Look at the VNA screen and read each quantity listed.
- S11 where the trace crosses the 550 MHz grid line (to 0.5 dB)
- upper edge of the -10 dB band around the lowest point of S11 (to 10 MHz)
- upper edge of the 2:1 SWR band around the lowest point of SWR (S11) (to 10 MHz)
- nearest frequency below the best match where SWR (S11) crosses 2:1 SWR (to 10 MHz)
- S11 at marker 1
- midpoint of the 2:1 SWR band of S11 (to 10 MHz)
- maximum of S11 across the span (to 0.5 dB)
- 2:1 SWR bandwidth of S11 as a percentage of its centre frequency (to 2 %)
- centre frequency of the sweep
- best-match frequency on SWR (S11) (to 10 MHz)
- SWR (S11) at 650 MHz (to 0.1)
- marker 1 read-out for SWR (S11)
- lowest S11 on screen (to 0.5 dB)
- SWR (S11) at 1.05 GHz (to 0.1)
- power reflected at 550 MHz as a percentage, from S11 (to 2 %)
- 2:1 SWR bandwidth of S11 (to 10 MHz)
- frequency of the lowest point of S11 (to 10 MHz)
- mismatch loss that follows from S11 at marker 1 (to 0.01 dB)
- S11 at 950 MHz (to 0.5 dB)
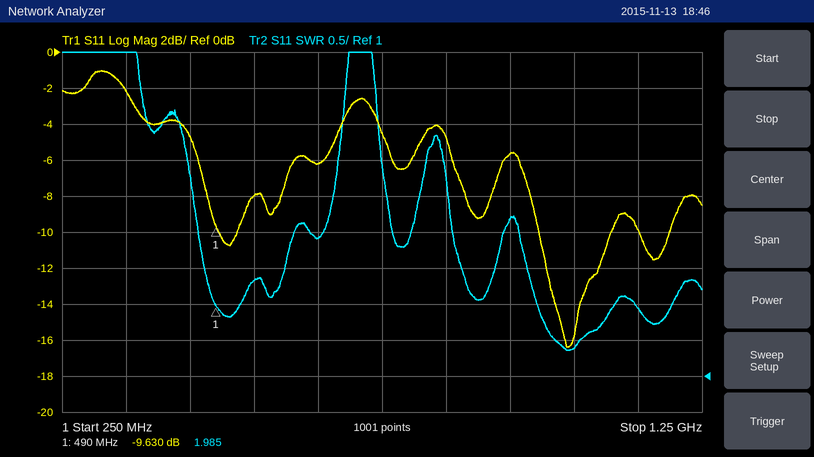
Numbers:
-8.0 dB
1.11 GHz
1.11 GHz
990 MHz
-9.630 dB
1.05 GHz
-1.0 dB
12 %
750 MHz
1.04 GHz
2.9
1.985
-16.5 dB
1.4
16 %
120 MHz
1.04 GHz
0.50 dB
-5.5 dB
